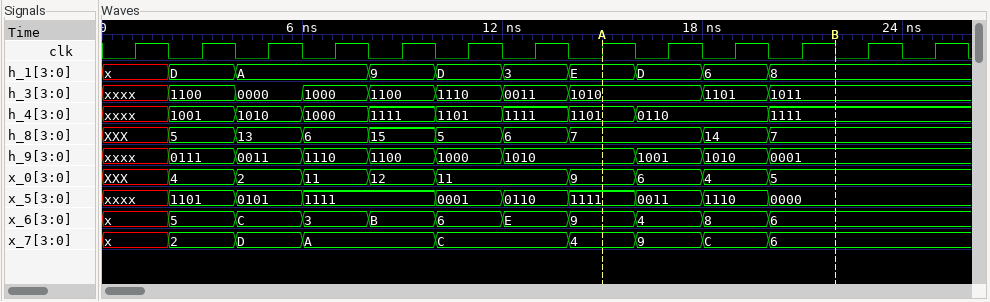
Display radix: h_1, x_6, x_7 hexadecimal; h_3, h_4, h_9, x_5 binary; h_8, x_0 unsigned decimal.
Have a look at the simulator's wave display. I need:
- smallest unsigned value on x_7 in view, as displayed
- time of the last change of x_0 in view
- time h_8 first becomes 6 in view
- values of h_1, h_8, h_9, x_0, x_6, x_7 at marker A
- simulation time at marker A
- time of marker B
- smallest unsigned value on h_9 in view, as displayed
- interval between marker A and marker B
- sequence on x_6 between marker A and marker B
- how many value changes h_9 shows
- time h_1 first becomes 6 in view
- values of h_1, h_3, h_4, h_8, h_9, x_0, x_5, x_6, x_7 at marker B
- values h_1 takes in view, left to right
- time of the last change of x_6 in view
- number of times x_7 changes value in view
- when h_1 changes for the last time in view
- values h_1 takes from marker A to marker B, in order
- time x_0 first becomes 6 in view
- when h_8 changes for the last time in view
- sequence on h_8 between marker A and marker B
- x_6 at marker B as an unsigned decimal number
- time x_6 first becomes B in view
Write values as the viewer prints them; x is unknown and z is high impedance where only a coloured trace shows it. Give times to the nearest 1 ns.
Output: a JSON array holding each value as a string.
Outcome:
["2", "20 ns", "6 ns", "h_1=E, h_8=7, h_9=1010, x_0=9, x_6=9, x_7=4", "15 ns", "22 ns", "0001", "7 ns", "9, 4, 8, 6", "9", "18 ns", "h_1=8, h_3=1011, h_4=1111, h_8=7, h_9=0001, x_0=5, x_5=0000, x_6=6, x_7=6", "x, D, A, 9, D, 3, E, D, 6, 8", "20 ns", "8", "20 ns", "E, D, 6, 8", "16 ns", "20 ns", "7, 14, 7", "6", "8 ns"]
